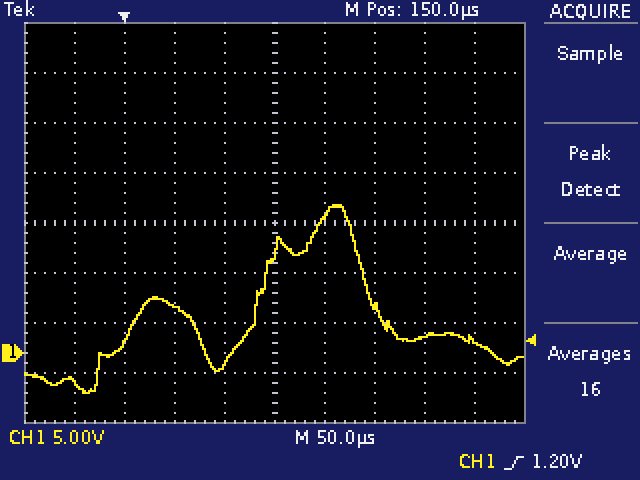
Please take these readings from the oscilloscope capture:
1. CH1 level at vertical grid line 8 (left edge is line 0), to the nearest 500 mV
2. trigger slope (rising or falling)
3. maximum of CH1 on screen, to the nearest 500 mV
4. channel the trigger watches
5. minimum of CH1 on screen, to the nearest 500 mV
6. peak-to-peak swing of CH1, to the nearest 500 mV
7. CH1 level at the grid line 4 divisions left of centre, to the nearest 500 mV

1.5 V
rising
15.0 V
CH1
-4.0 V
19.0 V
-3.0 V
